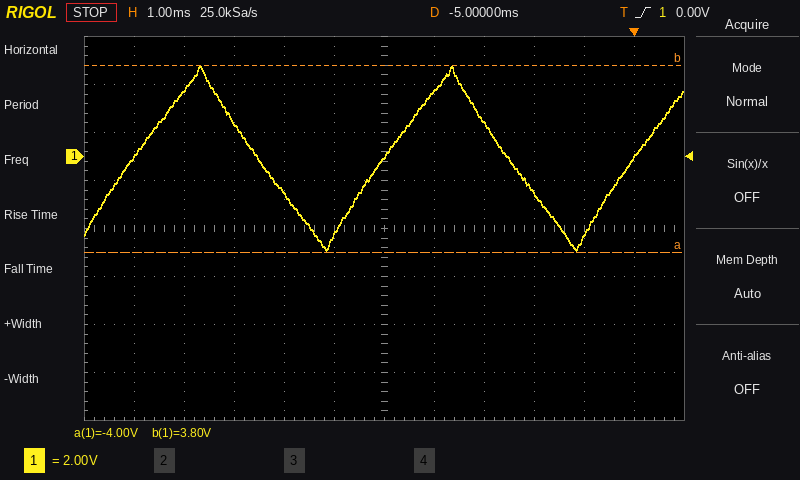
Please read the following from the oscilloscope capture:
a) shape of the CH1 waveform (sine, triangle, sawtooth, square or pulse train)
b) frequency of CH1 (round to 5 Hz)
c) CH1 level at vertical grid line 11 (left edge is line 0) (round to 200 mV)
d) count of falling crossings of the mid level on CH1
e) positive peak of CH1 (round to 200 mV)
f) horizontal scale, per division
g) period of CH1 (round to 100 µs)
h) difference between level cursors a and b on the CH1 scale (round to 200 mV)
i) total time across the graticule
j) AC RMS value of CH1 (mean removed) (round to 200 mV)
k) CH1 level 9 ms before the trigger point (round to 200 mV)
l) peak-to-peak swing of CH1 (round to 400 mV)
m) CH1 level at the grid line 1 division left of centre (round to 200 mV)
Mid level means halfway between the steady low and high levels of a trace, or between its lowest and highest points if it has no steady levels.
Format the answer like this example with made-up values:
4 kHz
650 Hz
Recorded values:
triangle
200 Hz
0.0 V
2
3.8 V
1 ms
5.0 ms
7.8 V
12 ms
2.2 V
2.8 V
7.6 V
-3.2 V
